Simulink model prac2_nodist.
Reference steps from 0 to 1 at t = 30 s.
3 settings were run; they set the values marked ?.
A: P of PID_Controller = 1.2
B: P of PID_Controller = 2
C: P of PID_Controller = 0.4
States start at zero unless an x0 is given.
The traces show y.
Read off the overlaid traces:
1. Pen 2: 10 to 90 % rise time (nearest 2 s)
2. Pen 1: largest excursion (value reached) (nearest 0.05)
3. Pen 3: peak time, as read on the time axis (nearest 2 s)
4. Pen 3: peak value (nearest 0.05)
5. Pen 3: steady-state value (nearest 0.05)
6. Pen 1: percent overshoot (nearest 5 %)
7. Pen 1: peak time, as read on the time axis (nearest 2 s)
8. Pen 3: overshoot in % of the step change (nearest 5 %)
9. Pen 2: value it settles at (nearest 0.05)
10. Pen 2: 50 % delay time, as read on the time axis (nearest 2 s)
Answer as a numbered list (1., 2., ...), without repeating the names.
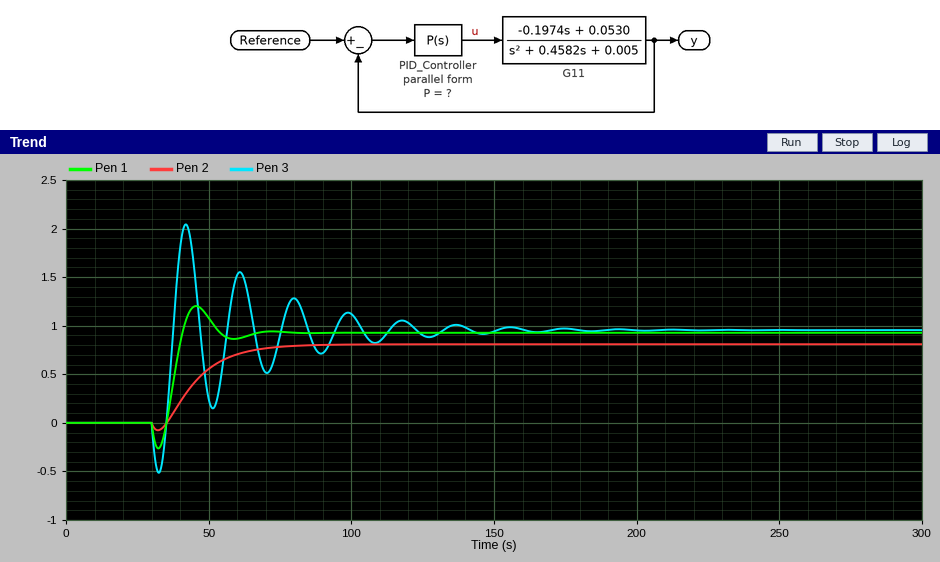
1. 26 s
2. 1.20
3. 42 s
4. 2.05
5. 0.95
6. 30 %
7. 46 s
8. 115 %
9. 0.80
10. 44 s
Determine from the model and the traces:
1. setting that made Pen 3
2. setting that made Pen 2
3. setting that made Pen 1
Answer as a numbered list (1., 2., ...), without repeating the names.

1. B
2. C
3. A
